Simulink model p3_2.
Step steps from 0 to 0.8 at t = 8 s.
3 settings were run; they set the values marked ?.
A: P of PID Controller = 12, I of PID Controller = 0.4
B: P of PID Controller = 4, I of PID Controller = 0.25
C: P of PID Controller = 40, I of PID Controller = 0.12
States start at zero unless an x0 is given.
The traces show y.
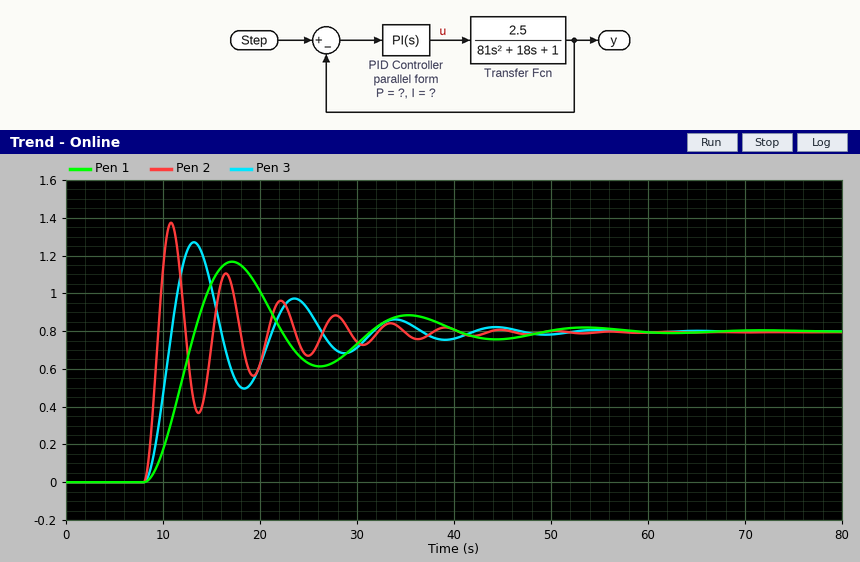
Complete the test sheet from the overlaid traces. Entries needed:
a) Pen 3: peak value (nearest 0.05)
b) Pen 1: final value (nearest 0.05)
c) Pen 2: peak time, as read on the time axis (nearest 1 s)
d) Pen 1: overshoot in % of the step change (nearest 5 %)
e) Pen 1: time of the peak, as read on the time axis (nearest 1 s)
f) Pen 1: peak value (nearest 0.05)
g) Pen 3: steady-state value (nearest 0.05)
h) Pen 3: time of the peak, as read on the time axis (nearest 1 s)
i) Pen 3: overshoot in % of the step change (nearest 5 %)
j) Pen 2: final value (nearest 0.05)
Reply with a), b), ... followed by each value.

a) 1.25
b) 0.80
c) 11 s
d) 45 %
e) 17 s
f) 1.15
g) 0.80
h) 13 s
i) 60 %
j) 0.80
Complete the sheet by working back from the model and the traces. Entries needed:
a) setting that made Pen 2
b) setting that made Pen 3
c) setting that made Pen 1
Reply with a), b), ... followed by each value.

a) C
b) A
c) B
